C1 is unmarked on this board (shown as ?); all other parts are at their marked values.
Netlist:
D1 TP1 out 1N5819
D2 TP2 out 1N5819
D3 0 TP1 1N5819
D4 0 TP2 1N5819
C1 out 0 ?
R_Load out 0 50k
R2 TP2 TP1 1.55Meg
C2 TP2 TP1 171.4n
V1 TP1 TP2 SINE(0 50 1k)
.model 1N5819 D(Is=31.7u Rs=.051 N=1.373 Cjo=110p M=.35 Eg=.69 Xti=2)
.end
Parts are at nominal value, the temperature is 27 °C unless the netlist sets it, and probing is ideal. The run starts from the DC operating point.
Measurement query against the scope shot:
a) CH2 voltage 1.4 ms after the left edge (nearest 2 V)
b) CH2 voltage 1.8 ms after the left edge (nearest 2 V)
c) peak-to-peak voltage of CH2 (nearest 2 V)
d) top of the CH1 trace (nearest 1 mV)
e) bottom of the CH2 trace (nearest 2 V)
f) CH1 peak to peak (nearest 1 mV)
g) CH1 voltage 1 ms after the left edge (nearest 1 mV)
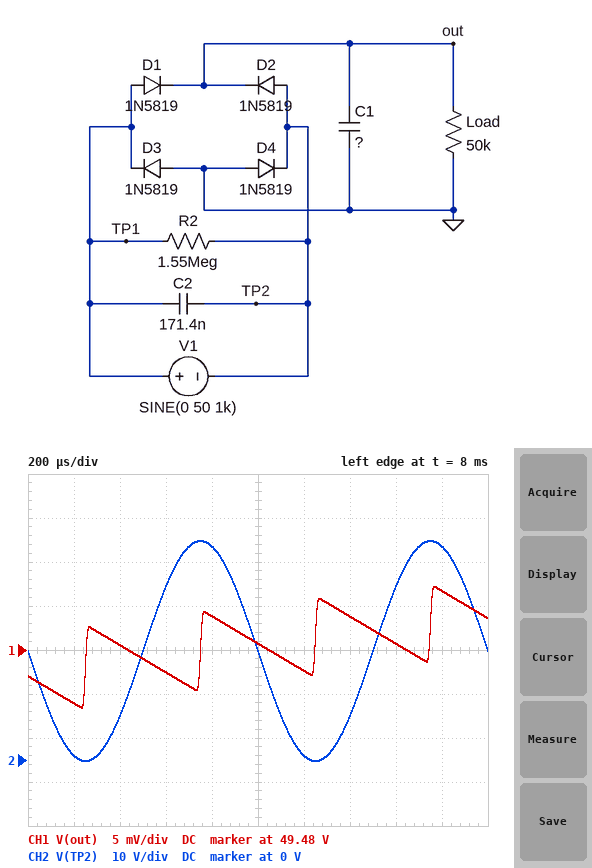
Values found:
10 V
48 V
50 V
49.492 V
0 V
14 mV
49.486 V
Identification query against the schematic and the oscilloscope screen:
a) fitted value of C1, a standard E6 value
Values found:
68 µF
